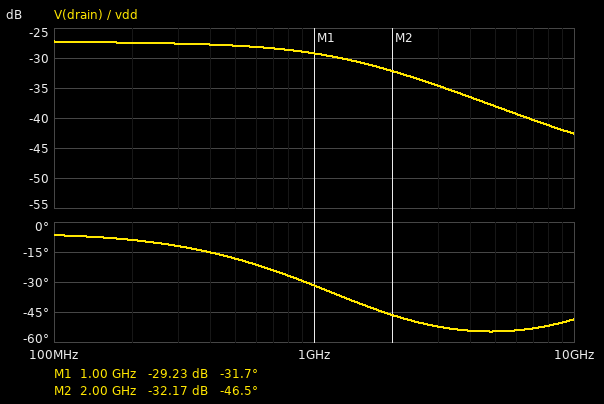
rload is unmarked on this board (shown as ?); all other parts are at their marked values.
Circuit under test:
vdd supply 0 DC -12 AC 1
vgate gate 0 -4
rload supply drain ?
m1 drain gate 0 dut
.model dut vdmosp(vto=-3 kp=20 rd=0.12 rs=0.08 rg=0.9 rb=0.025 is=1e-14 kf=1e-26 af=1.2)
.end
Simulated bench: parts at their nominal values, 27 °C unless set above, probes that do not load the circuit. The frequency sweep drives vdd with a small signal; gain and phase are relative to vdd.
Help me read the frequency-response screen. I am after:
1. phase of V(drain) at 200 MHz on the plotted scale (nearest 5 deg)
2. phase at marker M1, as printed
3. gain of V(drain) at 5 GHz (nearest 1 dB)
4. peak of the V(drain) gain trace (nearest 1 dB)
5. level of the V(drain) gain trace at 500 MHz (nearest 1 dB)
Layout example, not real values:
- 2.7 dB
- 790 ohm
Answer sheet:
- -10 deg
- -31.7 deg
- -38 dB
- -27 dB
- -28 dB
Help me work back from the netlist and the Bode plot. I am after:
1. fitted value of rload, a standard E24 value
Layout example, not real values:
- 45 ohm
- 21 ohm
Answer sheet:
- 5.6 Ω
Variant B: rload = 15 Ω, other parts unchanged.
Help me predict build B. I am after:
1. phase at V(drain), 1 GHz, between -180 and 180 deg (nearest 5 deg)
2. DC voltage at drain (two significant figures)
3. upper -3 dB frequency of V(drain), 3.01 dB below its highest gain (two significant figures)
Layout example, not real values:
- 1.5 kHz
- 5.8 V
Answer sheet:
- -35 deg
- -200 mV
- 1.1 GHz
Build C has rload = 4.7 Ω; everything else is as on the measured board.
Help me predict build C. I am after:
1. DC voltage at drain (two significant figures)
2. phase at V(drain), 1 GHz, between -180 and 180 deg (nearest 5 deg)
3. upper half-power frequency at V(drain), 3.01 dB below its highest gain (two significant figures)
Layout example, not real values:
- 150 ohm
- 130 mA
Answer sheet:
- -650 mV
- -30 deg
- 950 MHz
